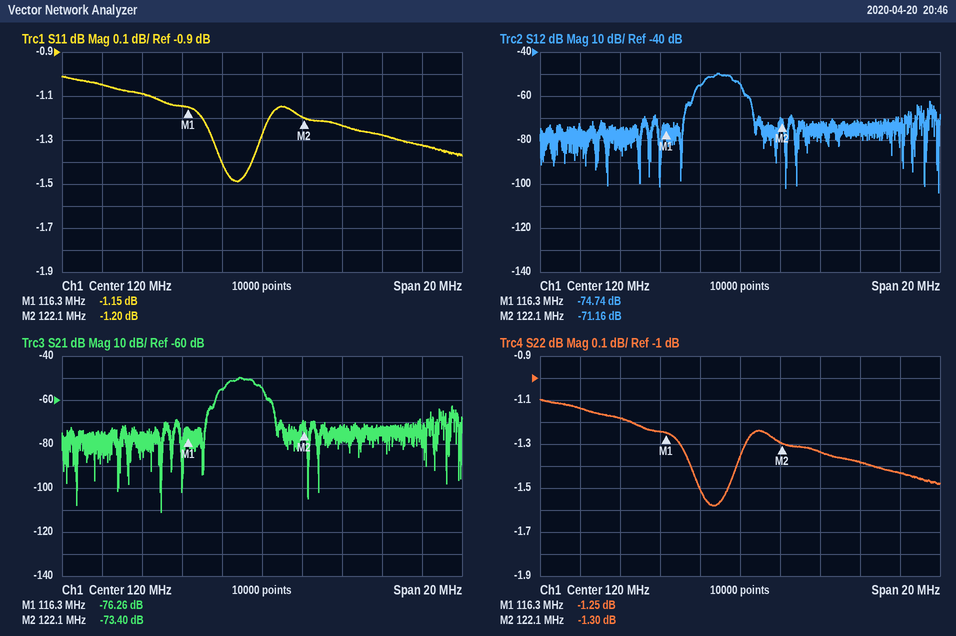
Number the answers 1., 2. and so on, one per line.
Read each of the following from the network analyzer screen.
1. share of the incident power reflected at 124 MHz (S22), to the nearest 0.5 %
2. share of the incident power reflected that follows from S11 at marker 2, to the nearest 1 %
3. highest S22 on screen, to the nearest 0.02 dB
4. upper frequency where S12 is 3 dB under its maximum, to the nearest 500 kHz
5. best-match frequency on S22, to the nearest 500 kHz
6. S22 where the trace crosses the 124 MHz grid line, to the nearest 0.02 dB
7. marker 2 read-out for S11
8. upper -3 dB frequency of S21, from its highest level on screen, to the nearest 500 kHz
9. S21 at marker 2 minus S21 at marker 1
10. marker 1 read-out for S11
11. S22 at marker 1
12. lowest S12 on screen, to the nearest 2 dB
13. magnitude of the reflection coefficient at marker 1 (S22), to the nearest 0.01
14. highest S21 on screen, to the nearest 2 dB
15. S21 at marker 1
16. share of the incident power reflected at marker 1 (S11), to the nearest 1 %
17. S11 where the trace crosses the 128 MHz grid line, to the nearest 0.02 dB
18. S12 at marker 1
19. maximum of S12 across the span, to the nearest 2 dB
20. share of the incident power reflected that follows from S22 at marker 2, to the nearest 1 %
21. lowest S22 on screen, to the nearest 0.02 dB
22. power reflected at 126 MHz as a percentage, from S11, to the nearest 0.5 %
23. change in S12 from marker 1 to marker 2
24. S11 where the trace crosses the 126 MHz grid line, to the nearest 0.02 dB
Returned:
1. 73.5 %
2. 76 %
3. -1.10 dB
4. 119.5 MHz
5. 118.5 MHz
6. -1.34 dB
7. -1.20 dB
8. 119.5 MHz
9. 2.86 dB
10. -1.15 dB
11. -1.25 dB
12. -104 dB
13. 0.87
14. -50 dB
15. -76.26 dB
16. 77 %
17. -1.32 dB
18. -74.74 dB
19. -50 dB
20. 74 %
21. -1.58 dB
22. 74.5 %
23. 3.58 dB
24. -1.28 dB
